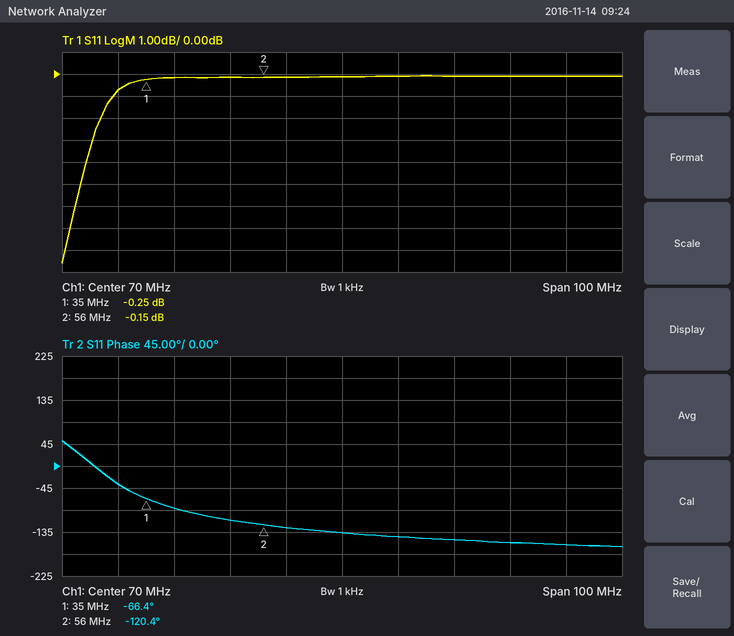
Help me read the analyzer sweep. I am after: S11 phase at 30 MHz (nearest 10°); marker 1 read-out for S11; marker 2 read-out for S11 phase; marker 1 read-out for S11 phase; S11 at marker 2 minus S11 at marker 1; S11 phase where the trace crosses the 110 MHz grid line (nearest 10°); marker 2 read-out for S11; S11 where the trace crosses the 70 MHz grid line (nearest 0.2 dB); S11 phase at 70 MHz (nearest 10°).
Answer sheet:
-40°
-0.25 dB
-120.4°
-66.4°
0.10 dB
-160°
-0.15 dB
-0.2 dB
-140°
